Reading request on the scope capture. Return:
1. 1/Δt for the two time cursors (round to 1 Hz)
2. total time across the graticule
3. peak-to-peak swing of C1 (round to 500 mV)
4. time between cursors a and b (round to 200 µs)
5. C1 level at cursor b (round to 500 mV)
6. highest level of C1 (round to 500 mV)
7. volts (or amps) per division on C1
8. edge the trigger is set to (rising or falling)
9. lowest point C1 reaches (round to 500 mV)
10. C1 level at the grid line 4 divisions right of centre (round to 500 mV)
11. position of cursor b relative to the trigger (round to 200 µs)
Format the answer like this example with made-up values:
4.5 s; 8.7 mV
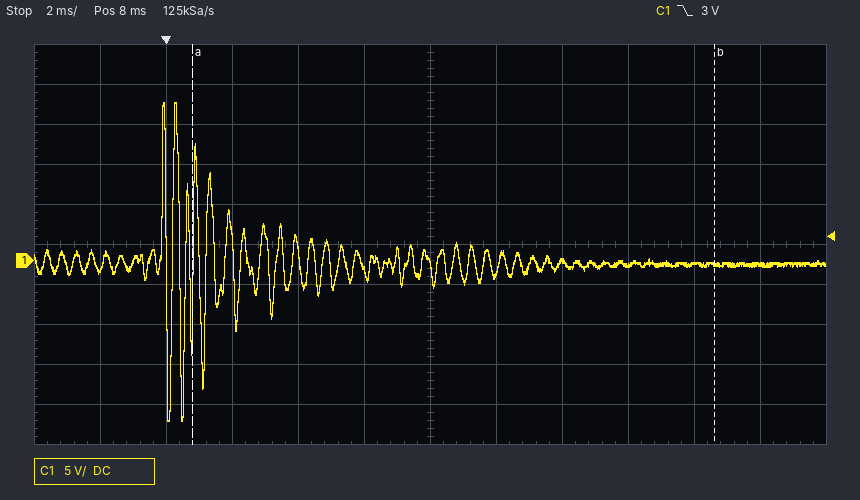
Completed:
63 Hz; 24 ms; 40.0 V; 15.8 ms; -500 mV; 20.0 V; 5 V; falling; -20.0 V; -500 mV; +16.6 ms
